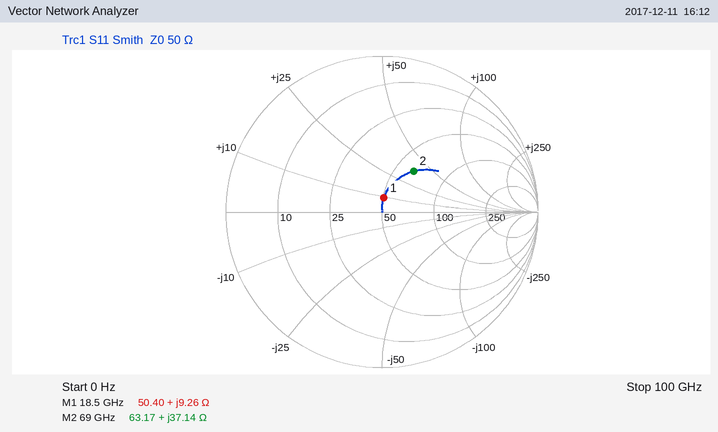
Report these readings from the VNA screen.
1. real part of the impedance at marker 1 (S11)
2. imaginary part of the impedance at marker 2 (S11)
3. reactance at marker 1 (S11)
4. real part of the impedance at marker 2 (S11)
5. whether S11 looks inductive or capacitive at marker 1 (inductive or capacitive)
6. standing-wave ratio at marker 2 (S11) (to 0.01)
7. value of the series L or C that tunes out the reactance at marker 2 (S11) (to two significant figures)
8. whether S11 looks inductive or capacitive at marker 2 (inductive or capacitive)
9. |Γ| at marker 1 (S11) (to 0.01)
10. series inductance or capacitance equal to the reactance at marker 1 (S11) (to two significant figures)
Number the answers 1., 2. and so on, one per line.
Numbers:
1. 50.40 Ω
2. +37.14 Ω
3. +9.26 Ω
4. 63.17 Ω
5. inductive
6. 1.99
7. 62 fF
8. inductive
9. 0.09
10. 80 pH
